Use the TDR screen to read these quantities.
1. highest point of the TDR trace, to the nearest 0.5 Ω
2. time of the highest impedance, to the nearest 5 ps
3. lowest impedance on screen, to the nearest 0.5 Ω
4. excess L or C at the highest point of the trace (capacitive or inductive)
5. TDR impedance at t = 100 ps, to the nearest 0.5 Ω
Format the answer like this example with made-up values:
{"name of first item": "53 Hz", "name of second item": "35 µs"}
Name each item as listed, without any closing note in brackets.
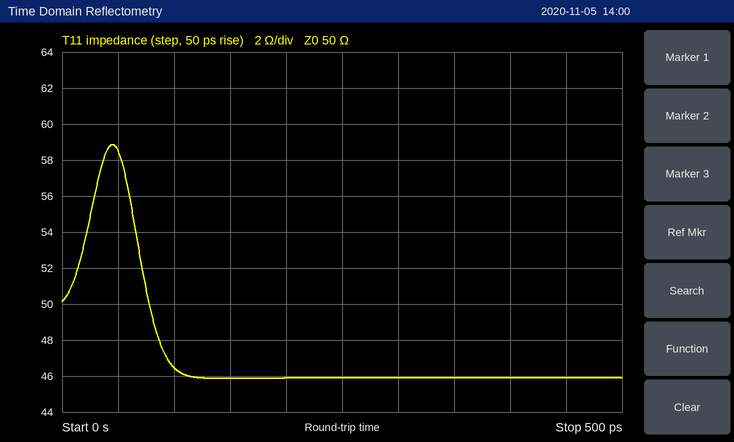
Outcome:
{"highest point of the TDR trace, to the nearest 0.5 Ω": "59.0 Ω", "time of the highest impedance, to the nearest 5 ps": "45 ps", "lowest impedance on screen, to the nearest 0.5 Ω": "46.0 Ω", "excess L or C at the highest point of the trace": "inductive", "TDR impedance at t = 100 ps, to the nearest 0.5 Ω": "46.5 Ω"}
